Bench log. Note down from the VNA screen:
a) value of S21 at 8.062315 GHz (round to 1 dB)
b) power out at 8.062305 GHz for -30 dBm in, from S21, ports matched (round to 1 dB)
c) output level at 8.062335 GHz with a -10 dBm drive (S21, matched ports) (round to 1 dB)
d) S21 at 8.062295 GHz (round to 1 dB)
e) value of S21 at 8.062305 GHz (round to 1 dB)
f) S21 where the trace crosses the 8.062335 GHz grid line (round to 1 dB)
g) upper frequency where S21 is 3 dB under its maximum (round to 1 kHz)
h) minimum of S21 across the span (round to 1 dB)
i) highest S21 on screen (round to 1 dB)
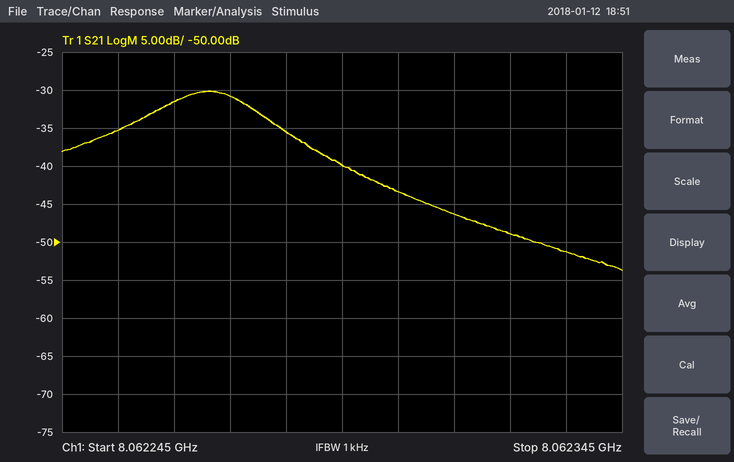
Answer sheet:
-46 dB
-73 dBm
-61 dBm
-40 dB
-43 dB
-51 dB
8.062280 GHz
-54 dB
-30 dB
